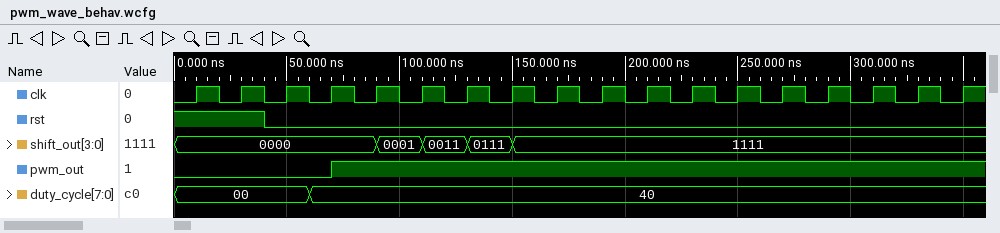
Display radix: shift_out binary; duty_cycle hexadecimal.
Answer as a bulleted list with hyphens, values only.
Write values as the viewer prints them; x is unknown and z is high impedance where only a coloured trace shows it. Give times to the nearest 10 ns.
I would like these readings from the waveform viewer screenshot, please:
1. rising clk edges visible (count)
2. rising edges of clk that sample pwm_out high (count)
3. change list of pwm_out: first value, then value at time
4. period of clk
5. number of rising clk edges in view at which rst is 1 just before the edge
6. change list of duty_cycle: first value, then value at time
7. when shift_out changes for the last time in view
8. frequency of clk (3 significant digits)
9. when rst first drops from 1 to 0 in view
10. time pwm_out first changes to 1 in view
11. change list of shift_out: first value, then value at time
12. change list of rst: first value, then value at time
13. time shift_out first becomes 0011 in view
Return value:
- 18
- 14
- 0, 1 at 70 ns
- 20 ns
- 2
- 00, 40 at 60 ns
- 150 ns
- 50.0 MHz
- 40 ns
- 70 ns
- 0000, 0001 at 90 ns, 0011 at 110 ns, 0111 at 130 ns, 1111 at 150 ns
- 1, 0 at 40 ns
- 110 ns
